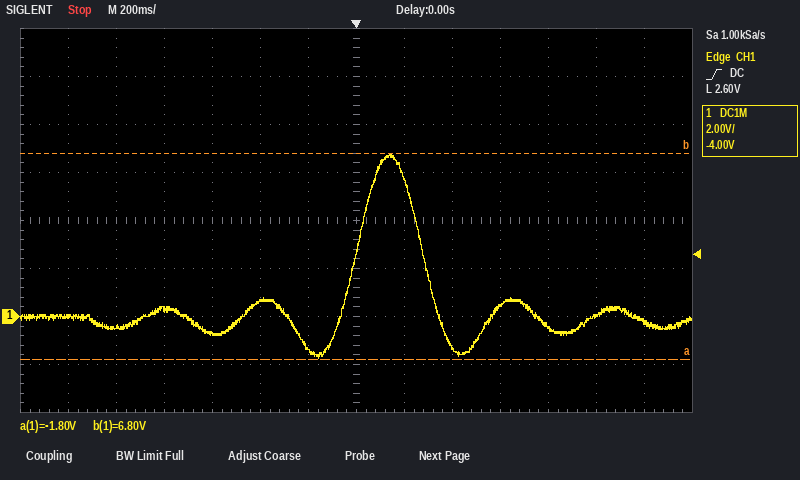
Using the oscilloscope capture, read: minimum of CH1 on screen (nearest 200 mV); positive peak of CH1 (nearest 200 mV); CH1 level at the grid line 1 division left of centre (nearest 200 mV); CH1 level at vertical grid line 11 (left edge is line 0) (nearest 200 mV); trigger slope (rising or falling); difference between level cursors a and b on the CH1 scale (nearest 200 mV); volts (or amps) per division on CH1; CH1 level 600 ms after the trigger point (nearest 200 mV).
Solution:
-1.8 V
6.8 V
-1.4 V
-400 mV
rising
8.6 V
2 V
400 mV
